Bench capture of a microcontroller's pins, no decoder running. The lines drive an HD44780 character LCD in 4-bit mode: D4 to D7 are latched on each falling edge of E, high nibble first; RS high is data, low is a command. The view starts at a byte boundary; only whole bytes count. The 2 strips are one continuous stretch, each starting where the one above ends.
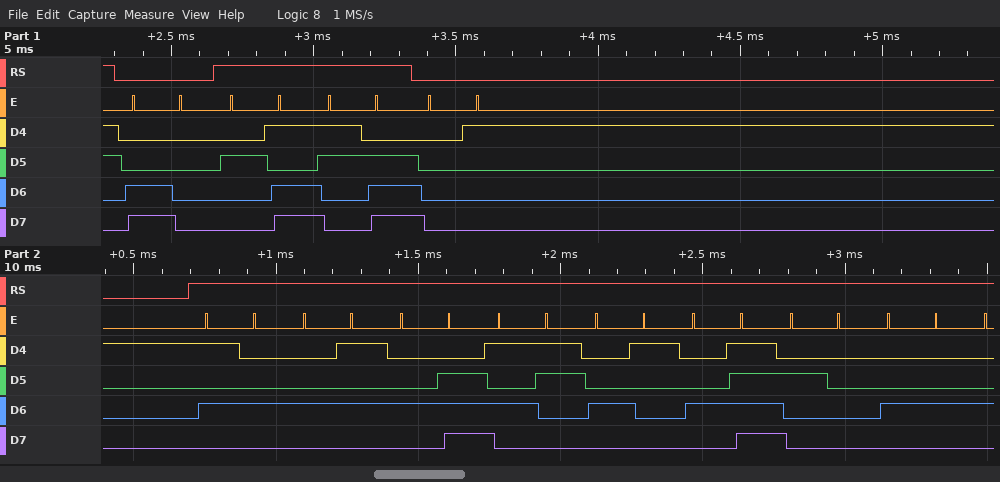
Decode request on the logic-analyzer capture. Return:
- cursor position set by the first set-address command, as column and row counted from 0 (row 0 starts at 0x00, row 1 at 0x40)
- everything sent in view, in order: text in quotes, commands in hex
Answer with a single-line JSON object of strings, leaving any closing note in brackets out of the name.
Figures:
{"cursor position set by the first set-address command, as column and row counted from 0": "column 0, row 1", "everything sent in view, in order: text in quotes, commands in hex": "0xC0 \"->\" 0x01 \"TENSAO D\""}
